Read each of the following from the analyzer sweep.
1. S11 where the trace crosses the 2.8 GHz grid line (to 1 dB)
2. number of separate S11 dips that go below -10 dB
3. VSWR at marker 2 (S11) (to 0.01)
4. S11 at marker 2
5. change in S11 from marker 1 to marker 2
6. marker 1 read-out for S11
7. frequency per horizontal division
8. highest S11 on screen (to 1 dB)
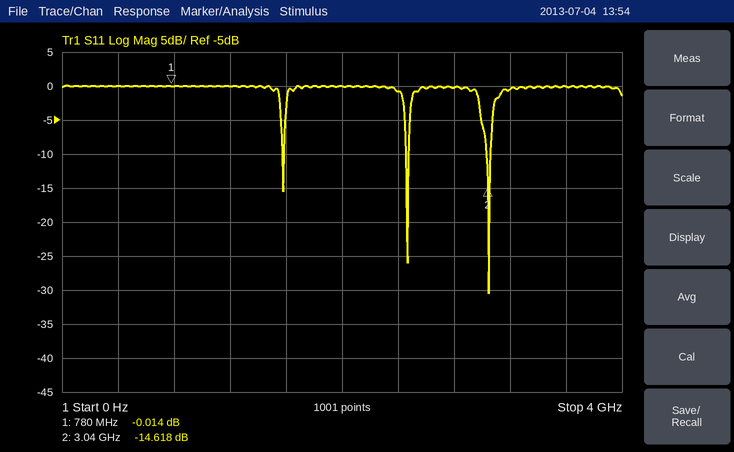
0 dB
3
1.46
-14.618 dB
-14.604 dB
-0.014 dB
400 MHz
0 dB
